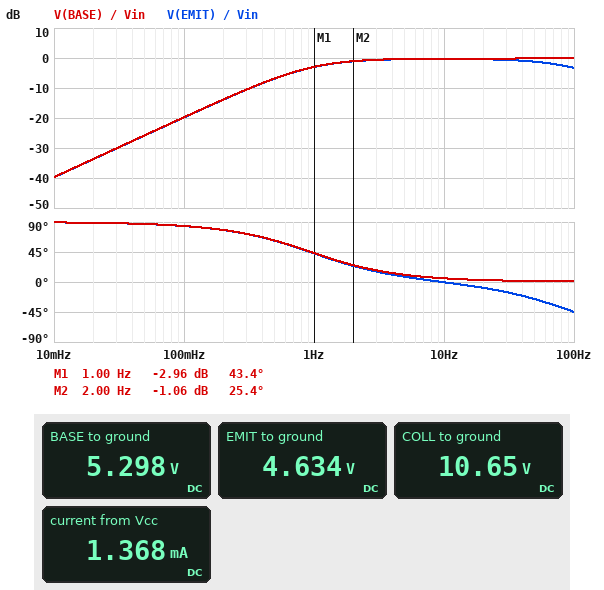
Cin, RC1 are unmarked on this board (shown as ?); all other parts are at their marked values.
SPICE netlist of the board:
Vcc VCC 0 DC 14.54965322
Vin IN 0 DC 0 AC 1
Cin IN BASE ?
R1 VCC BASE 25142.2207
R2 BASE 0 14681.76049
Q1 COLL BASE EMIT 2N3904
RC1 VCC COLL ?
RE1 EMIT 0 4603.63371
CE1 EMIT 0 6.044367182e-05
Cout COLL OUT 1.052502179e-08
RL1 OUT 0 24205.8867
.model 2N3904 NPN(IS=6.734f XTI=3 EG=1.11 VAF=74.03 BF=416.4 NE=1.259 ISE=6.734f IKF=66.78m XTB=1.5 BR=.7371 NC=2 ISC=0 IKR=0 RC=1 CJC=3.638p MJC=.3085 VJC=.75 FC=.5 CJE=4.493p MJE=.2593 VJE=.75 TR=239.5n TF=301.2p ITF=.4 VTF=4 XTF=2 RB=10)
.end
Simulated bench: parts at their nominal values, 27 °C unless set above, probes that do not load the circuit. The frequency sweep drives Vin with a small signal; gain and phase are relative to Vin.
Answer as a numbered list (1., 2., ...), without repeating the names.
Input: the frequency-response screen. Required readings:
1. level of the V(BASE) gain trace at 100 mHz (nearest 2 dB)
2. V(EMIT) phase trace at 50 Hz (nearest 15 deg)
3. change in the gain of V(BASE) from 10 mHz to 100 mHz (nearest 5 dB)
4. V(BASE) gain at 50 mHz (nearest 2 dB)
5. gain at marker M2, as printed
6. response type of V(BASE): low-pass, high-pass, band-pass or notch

1. -20 dB
2. -30 deg
3. 20 dB
4. -26 dB
5. -1.06 dB
6. high-pass
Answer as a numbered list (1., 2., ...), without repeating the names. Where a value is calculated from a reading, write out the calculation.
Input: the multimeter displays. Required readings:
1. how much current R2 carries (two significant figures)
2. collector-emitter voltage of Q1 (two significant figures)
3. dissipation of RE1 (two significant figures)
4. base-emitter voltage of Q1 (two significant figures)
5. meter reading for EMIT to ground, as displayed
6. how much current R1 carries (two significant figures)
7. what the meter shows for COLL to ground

1. (5.298 V) / 14.68 kΩ = 360 µA
2. 10.65 V - 4.634 V = 6.0 V
3. (4.634 V)^2 / 4.604 kΩ = 4.7 mW
4. 5.298 V - 4.634 V = 660 mV
5. 4.634 V
6. (14.55 V - 5.298 V) / 25.14 kΩ = 370 µA
7. 10.65 V
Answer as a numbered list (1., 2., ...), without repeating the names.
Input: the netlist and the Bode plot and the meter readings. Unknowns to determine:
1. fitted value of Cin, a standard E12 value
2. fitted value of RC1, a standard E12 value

1. 18 µF
2. 3.9 kΩ
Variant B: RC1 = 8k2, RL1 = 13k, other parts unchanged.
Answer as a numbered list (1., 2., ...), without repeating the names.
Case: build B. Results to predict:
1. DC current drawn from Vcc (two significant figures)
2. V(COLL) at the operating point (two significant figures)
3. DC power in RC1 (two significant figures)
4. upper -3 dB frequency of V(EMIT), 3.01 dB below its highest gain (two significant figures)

1. 1.4 mA
2. 6.4 V
3. 8.2 mW
4. 95 Hz
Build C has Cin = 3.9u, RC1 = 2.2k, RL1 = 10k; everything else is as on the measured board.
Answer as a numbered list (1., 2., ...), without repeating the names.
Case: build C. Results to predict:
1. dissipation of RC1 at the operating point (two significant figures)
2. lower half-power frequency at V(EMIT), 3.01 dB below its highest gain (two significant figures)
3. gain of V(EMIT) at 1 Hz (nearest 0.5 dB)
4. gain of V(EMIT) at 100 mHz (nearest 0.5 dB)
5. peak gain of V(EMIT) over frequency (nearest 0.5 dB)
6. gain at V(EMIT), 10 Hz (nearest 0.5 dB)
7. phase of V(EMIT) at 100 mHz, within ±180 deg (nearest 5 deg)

1. 2.2 mW
2. 3.8 Hz
3. -13.5 dB
4. -33.0 dB
5. -1.0 dB
6. -1.5 dB
7. 90 deg
